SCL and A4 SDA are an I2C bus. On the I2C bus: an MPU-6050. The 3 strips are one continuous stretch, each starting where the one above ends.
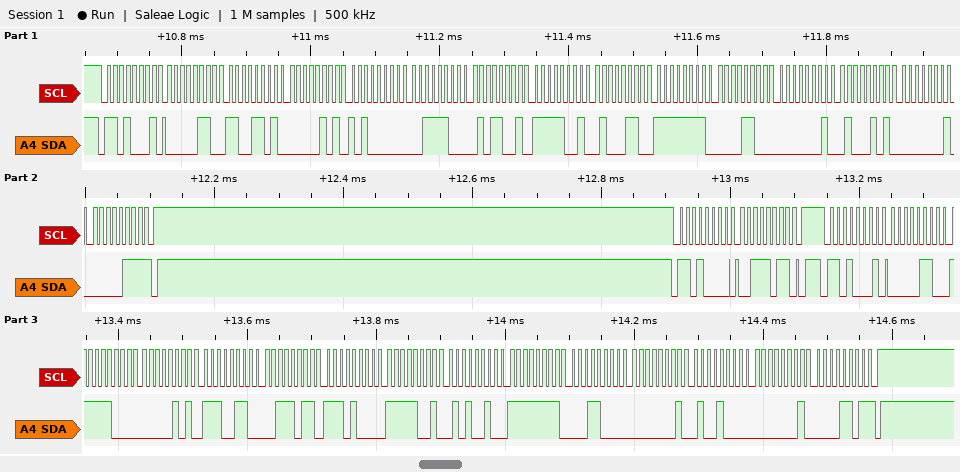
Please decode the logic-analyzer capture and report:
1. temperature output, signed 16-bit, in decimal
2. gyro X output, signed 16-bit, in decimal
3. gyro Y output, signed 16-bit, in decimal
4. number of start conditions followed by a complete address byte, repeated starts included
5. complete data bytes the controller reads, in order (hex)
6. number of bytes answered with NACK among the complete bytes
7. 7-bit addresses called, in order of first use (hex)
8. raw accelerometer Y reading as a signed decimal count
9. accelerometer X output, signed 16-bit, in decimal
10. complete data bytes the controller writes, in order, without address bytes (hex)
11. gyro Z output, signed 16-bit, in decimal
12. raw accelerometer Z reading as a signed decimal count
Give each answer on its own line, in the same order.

-1710
-232
328
3
06 CD 05 A0 3C 59 F9 46 FF 0C 01 45 01 07 06 F8 05 E6 3B E8 F9 52 FF 18 01 48 01 0D
2
0x68
1510
1784
3B
269
15336
